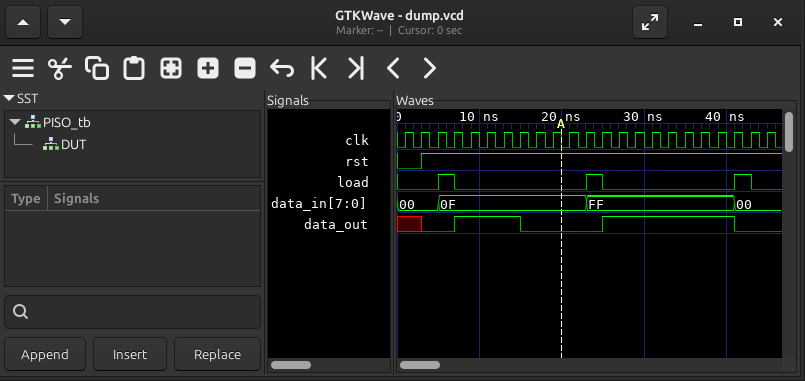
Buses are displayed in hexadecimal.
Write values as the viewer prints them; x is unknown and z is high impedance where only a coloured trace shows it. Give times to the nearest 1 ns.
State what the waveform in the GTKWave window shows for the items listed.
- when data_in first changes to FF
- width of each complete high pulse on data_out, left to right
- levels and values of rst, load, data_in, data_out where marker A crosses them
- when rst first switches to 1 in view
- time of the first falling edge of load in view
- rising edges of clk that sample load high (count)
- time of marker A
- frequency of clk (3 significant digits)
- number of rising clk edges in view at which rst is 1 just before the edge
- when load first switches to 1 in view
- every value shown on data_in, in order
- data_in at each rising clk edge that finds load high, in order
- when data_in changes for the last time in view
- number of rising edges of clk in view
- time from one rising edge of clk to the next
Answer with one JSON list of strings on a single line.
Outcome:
["23 ns", "8 ns, 16 ns", "rst=1, load=0, data_in=0F, data_out=0", "3 ns", "7 ns", "3", "20 ns", "500 MHz", "21", "5 ns", "00, 0F, FF, 00", "0F, FF, 00", "41 ns", "23", "2 ns"]
